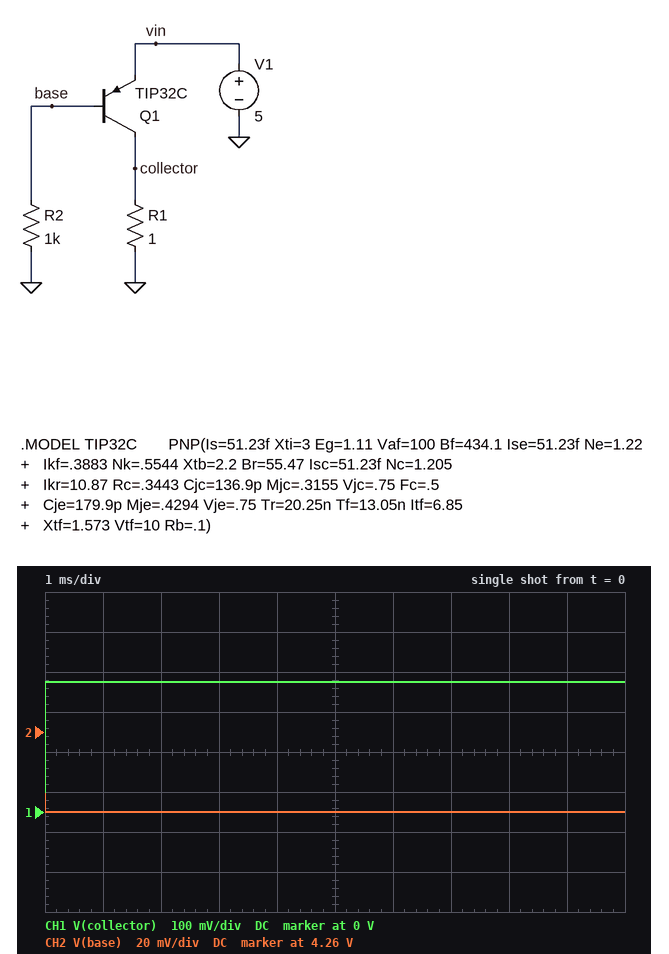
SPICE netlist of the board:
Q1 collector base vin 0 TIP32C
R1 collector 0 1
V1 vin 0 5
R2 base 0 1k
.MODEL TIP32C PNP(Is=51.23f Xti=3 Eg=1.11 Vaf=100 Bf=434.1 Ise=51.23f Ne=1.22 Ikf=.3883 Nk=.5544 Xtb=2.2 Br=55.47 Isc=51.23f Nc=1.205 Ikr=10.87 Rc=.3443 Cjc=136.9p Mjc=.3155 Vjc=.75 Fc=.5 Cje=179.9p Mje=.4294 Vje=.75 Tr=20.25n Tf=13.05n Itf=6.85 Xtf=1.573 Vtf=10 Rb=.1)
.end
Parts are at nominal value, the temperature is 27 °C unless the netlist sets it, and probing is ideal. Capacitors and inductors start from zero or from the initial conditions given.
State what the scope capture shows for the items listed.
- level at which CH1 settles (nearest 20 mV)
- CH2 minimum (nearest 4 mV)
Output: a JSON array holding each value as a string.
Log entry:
["320 mV", "4.220 V"]
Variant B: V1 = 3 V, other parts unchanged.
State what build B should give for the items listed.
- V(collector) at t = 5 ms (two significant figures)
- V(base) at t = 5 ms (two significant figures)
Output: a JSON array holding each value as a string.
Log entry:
["200 mV", "2.2 V"]
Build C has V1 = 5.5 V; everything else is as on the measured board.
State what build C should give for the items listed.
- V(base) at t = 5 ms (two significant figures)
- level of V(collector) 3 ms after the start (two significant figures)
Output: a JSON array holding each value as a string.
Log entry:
["4.7 V", "350 mV"]
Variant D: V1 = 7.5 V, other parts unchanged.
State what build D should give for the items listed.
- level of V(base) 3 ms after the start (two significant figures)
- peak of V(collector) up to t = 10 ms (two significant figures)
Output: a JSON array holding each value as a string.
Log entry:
["6.7 V", "460 mV"]
